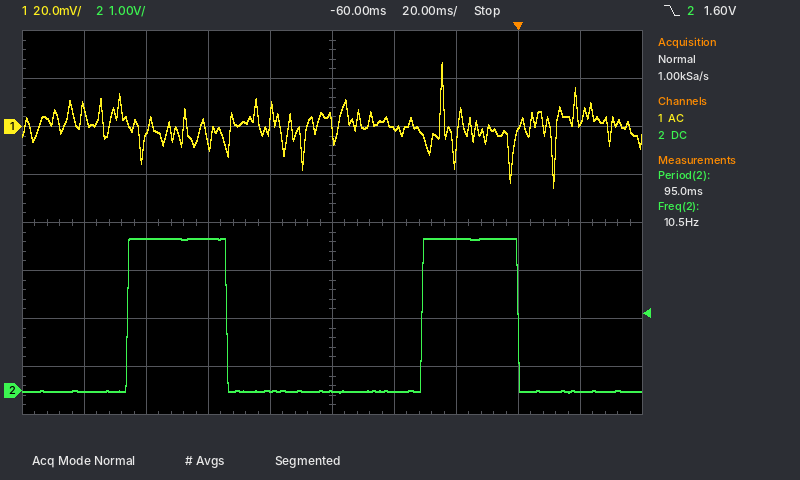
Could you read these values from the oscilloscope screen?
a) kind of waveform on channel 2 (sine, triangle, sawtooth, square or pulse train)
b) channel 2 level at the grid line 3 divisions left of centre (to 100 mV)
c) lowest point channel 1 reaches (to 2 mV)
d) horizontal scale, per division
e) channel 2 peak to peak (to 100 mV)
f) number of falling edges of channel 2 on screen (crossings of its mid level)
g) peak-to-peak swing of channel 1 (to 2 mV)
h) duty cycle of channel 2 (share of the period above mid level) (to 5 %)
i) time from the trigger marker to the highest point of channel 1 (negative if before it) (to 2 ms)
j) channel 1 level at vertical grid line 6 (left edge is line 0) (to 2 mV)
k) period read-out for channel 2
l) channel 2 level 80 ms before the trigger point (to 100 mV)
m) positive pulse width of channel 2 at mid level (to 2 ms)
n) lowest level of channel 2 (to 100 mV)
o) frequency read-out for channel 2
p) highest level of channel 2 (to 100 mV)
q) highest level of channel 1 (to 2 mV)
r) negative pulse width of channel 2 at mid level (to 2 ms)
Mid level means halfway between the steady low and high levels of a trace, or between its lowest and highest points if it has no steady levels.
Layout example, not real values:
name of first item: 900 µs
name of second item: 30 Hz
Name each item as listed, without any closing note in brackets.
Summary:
kind of waveform on channel 2: pulse train
channel 2 level at the grid line 3 divisions left of centre: 3.2 V
lowest point channel 1 reaches: -26 mV
horizontal scale, per division: 20 ms
channel 2 peak to peak: 3.2 V
number of falling edges of channel 2 on screen: 2
peak-to-peak swing of channel 1: 52 mV
duty cycle of channel 2 (share of the period above mid level): 35 %
time from the trigger marker to the highest point of channel 1 (negative if before it): -24 ms
channel 1 level at vertical grid line 6 (left edge is line 0): 0 mV
period read-out for channel 2: 95.0 ms
channel 2 level 80 ms before the trigger point: 0.0 V
positive pulse width of channel 2 at mid level: 32 ms
lowest level of channel 2: 0.0 V
frequency read-out for channel 2: 10.5 Hz
highest level of channel 2: 3.2 V
highest level of channel 1: 26 mV
negative pulse width of channel 2 at mid level: 64 ms
